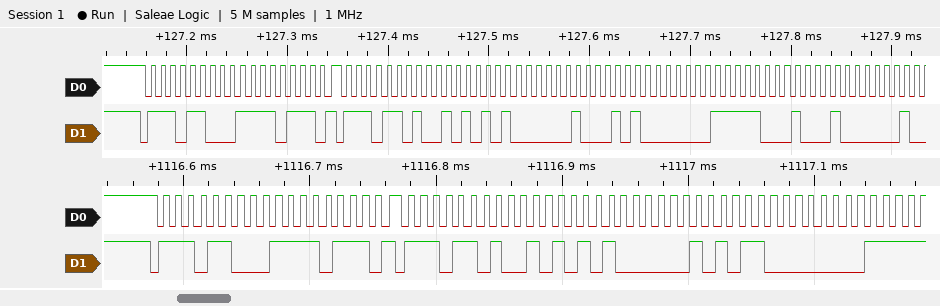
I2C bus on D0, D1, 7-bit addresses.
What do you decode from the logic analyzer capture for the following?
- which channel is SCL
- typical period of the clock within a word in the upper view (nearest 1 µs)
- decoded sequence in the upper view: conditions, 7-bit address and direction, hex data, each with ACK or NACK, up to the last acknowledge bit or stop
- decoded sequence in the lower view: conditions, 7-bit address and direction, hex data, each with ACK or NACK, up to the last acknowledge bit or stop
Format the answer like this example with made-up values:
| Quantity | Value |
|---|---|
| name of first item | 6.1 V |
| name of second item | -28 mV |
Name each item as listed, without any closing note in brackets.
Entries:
| Quantity | Value |
|---|---|
| which channel is SCL | D0 |
| typical period of the clock within a word in the upper view | 10 µs |
| decoded sequence in the upper view: conditions, 7-bit address and direction, hex data, each with ACK or NACK, up to the last acknowledge bit or stop | start, address 76 write ACK, F7 ACK, repeated start, address 76 read ACK, 55 ACK, 04 ACK, A0 ACK, 7C ACK, 88 ACK |
| decoded sequence in the lower view: conditions, 7-bit address and direction, hex data, each with ACK or NACK, up to the last acknowledge bit or stop | start, address 76 write ACK, F7 ACK, repeated start, address 76 read ACK, 55 ACK, 05 ACK, C0 ACK |
